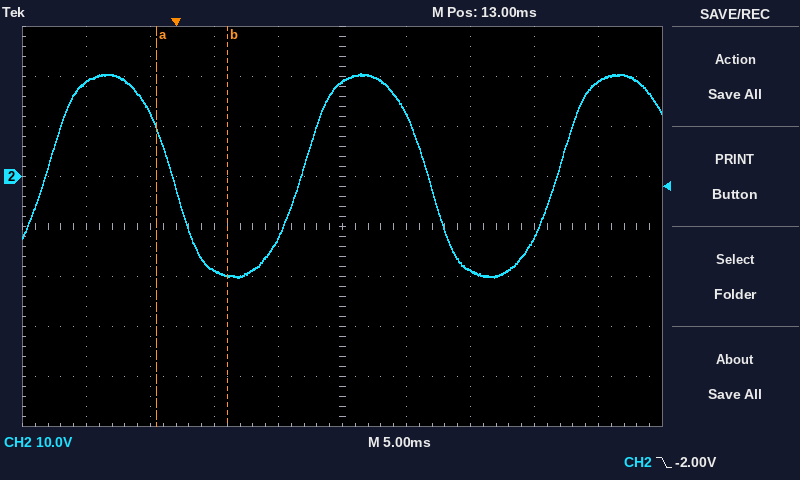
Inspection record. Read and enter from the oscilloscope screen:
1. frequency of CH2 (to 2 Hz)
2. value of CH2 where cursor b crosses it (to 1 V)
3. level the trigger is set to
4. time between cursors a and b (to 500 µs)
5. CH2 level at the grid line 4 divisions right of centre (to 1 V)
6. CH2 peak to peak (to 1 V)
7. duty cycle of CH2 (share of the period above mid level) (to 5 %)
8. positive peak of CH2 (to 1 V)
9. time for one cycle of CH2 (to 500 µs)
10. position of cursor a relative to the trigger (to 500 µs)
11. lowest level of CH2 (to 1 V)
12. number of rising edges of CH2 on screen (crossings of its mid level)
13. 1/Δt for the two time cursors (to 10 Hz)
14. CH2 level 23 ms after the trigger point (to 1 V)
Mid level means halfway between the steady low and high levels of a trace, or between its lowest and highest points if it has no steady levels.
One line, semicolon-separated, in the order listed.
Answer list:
50 Hz; -20 V; -2.00 V; 5.5 ms; 19 V; 41 V; 50 %; 21 V; 20.0 ms; -1.5 ms; -20 V; 3; 180 Hz; -19 V
